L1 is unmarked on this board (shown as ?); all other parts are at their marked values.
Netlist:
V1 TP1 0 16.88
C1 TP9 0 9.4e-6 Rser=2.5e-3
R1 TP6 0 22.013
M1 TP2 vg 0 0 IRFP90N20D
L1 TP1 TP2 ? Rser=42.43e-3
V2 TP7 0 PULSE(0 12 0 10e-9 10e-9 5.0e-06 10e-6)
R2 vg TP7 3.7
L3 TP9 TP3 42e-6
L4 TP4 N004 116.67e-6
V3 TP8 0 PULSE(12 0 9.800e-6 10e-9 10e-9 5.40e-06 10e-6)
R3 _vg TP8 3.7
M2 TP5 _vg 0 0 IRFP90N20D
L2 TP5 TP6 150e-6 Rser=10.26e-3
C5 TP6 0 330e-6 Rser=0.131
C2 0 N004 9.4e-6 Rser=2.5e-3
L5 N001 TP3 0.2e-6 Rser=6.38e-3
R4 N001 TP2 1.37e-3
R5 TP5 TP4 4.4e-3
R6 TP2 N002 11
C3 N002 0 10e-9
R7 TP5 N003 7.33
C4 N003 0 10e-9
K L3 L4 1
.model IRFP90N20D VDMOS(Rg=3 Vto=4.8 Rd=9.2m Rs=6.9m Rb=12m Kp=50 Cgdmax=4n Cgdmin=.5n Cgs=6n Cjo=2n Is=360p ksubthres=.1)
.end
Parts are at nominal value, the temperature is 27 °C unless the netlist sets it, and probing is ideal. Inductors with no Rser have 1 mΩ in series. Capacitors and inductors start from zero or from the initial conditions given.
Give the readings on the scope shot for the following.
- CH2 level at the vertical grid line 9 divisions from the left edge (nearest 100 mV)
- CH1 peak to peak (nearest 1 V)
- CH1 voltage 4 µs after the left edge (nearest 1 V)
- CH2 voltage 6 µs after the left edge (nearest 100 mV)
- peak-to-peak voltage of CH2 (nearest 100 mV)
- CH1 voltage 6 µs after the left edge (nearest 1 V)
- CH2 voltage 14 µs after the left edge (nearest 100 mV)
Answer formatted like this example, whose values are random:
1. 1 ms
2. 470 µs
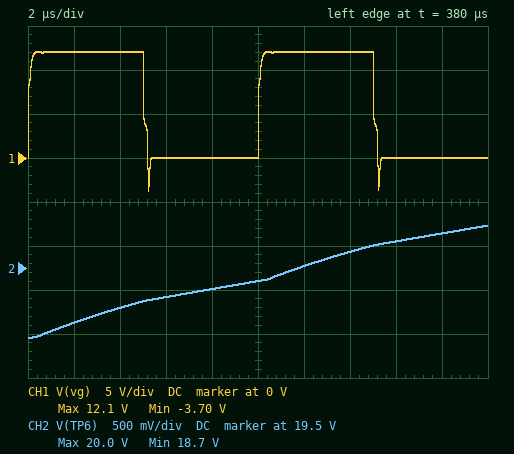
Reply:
1. 19.9 V
2. 16 V
3. 12 V
4. 19.2 V
5. 1.3 V
6. 0 V
7. 19.7 V
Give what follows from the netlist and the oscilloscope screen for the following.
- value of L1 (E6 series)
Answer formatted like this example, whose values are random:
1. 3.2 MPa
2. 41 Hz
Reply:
1. 33 µH
